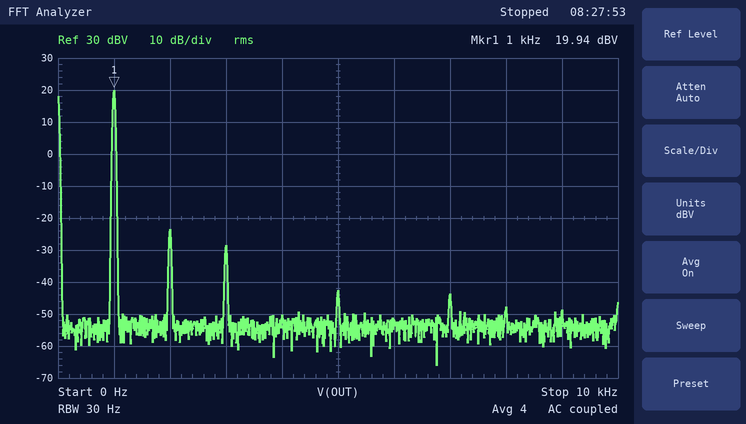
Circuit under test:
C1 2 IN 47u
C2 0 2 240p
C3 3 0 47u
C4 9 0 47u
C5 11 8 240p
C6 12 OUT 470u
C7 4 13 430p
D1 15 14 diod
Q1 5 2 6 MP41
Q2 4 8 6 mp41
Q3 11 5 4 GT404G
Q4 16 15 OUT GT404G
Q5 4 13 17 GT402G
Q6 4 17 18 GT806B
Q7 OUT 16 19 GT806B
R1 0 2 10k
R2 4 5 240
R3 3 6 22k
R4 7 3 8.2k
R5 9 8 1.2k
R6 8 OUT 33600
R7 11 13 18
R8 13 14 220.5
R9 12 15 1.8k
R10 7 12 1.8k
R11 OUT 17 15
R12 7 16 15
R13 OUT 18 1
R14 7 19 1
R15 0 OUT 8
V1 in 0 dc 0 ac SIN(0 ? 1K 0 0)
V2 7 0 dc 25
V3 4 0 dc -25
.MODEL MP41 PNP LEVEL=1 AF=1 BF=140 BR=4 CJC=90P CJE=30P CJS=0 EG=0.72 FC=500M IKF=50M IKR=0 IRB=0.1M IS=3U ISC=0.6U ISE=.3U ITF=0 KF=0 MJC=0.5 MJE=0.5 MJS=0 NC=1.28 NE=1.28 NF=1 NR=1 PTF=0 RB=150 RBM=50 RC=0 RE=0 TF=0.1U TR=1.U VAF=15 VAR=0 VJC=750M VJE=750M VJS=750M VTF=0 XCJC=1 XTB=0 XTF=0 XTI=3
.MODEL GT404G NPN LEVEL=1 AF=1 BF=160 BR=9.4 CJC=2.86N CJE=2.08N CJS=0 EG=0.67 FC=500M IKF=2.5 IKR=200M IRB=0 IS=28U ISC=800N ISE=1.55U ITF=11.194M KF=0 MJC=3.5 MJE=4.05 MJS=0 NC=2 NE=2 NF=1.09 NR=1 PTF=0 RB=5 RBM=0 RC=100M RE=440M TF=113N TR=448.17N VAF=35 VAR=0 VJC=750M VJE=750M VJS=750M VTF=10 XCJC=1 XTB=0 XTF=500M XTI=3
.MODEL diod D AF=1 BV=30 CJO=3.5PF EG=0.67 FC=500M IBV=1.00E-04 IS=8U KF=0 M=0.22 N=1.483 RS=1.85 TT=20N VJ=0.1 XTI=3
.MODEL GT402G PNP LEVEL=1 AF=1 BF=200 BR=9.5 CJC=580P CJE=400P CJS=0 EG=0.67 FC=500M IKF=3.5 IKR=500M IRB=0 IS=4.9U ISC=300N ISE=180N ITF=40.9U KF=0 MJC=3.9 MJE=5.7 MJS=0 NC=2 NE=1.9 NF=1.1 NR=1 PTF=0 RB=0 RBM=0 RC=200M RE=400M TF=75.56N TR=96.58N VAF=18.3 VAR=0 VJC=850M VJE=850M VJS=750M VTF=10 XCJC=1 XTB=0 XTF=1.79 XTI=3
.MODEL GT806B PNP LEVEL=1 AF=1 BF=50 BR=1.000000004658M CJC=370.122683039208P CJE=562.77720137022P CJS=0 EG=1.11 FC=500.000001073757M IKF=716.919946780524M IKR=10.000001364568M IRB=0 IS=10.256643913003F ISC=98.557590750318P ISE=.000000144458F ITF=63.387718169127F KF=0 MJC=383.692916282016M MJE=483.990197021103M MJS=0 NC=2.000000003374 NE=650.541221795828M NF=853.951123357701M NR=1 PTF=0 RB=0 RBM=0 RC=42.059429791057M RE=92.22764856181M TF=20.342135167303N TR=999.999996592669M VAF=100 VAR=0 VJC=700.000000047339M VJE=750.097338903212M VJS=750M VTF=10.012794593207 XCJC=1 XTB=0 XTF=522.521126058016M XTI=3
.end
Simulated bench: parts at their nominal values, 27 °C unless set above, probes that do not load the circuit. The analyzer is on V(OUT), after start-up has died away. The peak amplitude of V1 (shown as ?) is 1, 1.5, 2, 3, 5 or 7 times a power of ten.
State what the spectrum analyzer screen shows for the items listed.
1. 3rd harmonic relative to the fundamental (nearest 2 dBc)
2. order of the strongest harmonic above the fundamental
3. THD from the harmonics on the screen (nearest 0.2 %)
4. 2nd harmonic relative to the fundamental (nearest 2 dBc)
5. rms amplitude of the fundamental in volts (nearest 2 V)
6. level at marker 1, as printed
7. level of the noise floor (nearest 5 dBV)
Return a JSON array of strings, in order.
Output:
["-48 dBc", "2", "0.8 %", "-44 dBc", "10 V", "19.94 dBV", "-55 dBV"]
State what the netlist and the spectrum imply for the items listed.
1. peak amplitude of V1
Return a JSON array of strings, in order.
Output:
["500 mV"]
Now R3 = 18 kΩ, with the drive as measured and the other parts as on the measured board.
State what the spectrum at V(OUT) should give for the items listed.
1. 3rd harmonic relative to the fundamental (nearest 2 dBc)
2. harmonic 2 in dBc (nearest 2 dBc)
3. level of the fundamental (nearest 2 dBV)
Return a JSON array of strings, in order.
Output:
["-52 dBc", "-48 dBc", "20 dBV"]
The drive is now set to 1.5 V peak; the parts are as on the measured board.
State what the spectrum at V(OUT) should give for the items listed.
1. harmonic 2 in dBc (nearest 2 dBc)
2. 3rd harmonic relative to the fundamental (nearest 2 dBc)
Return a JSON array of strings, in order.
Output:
["-38 dBc", "-14 dBc"]
